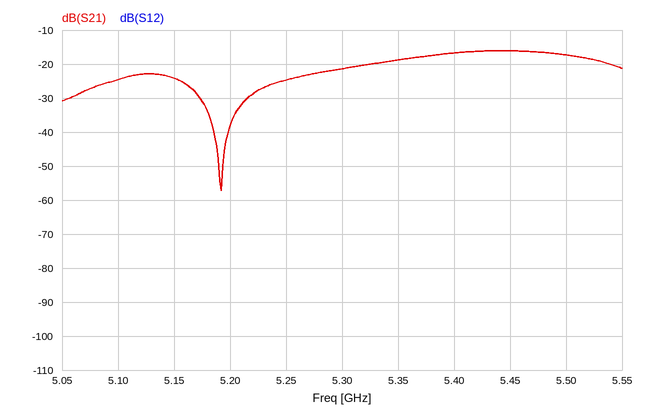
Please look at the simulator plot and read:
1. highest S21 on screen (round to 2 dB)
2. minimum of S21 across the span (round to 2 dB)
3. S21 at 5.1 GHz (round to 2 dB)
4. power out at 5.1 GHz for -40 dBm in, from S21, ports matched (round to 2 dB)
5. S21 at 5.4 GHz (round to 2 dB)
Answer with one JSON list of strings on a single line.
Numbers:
["-16 dB", "-58 dB", "-24 dB", "-64 dBm", "-16 dB"]
